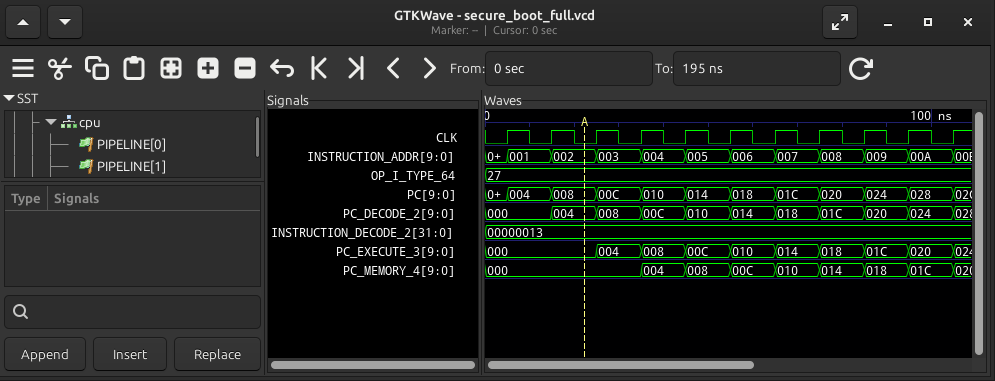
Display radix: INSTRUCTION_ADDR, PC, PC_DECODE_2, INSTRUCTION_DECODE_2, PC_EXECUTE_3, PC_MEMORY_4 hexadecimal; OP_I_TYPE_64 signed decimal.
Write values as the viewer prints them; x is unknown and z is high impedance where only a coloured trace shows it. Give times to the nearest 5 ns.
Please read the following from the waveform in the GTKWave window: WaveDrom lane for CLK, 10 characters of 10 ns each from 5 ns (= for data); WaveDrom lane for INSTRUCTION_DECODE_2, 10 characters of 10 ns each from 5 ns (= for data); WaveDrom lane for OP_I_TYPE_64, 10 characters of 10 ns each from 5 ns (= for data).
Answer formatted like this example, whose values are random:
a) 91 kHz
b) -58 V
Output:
a) {name: 'CLK', wave: 'p.........'}
b) {name: 'INSTRUCTION_DECODE_2', wave: '=.........', data: '00000013'}
c) {name: 'OP_I_TYPE_64', wave: '=.........', data: '27'}
